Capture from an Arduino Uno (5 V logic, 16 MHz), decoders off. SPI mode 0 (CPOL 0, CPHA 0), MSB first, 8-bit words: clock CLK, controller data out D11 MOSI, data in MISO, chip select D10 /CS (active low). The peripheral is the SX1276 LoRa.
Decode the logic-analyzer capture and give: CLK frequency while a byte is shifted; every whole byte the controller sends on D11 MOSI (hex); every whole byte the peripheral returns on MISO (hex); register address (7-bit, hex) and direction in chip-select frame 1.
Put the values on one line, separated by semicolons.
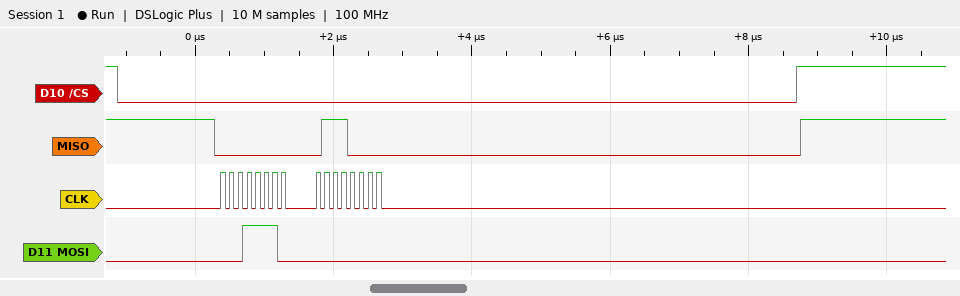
8 MHz; 1E 00; 00 70; 0x1E read
